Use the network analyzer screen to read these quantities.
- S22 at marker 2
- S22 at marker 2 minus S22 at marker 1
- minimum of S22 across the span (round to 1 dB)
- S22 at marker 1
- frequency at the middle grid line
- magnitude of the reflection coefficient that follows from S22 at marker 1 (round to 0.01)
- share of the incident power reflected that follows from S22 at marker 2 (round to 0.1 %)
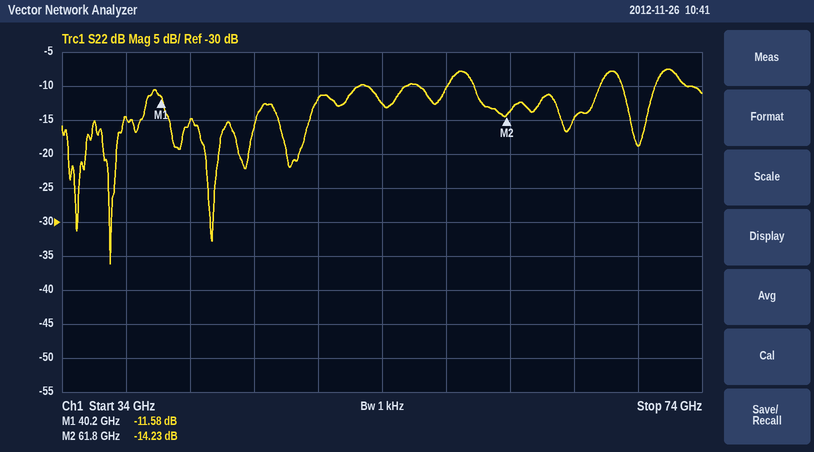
-14.23 dB
-2.65 dB
-36 dB
-11.58 dB
54 GHz
0.26
3.8 %
